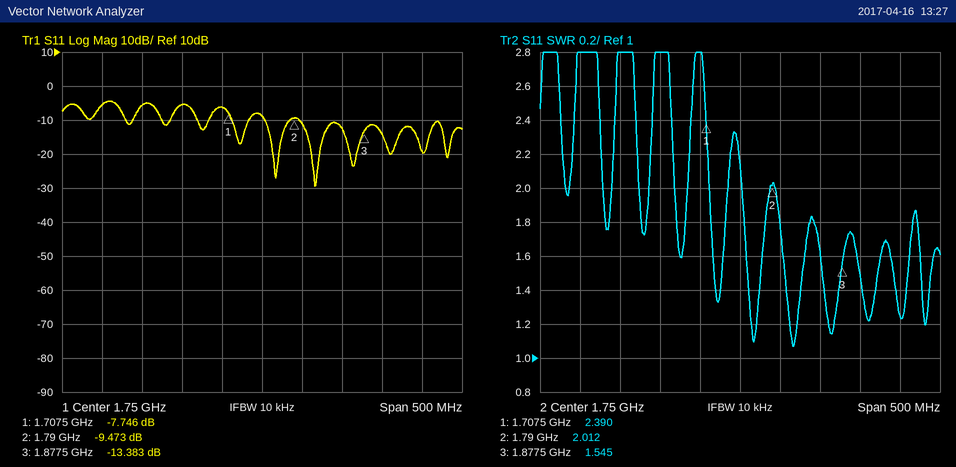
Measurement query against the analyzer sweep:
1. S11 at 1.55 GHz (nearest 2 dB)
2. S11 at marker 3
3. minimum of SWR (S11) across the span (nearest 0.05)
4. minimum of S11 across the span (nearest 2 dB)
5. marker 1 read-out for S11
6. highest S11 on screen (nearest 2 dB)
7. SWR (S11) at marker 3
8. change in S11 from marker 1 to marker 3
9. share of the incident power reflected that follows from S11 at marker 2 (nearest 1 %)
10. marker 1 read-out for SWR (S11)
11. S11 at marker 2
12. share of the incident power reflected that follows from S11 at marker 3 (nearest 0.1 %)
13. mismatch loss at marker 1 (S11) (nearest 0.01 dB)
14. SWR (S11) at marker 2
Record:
-6 dB
-13.383 dB
1.05
-30 dB
-7.746 dB
-4 dB
1.545
-5.637 dB
11 %
2.390
-9.473 dB
4.6 %
0.80 dB
2.012
